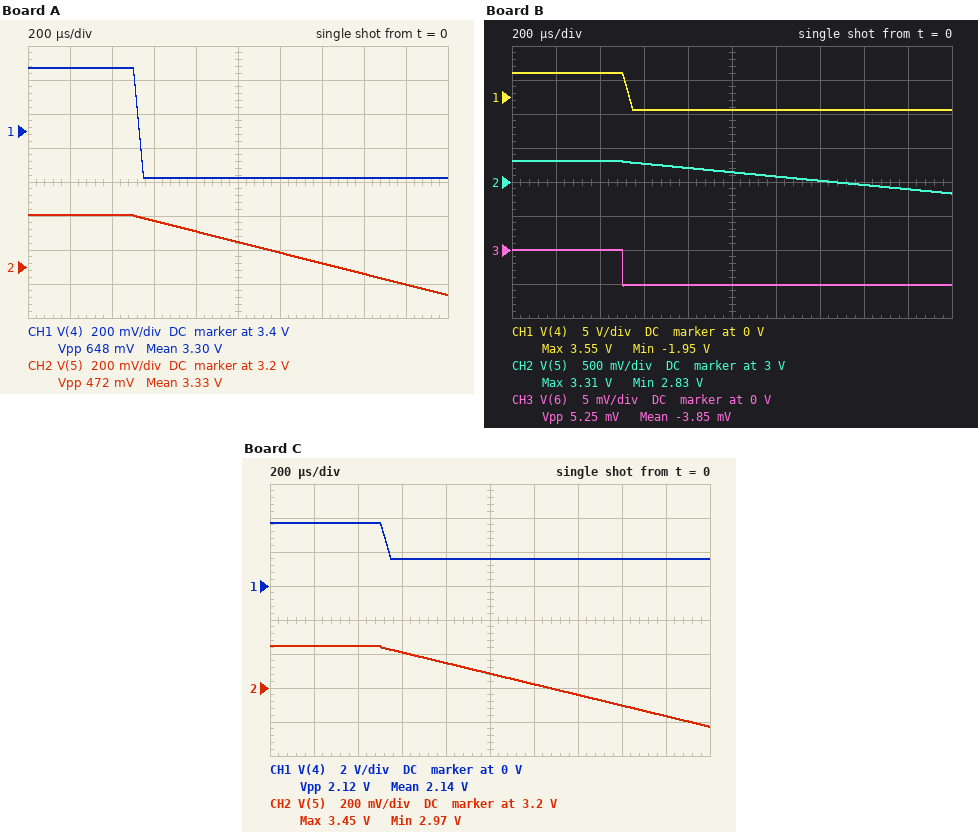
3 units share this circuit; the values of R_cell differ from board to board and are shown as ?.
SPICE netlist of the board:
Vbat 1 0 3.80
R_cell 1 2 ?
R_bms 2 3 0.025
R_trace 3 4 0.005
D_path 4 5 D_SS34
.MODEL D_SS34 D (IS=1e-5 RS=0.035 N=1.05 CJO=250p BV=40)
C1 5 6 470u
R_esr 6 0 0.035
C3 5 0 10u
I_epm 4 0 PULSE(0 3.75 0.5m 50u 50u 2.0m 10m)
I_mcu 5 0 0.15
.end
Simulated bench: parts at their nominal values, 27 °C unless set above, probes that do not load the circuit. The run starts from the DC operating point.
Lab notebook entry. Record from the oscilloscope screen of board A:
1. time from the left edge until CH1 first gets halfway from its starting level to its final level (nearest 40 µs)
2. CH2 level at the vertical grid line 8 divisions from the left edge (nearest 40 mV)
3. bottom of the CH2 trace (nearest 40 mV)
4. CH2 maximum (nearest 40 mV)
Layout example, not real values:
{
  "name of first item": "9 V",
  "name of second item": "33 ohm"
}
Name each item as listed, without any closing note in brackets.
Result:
{
  "time from the left edge until CH1 first gets halfway from its starting level to its final level": "520 µs",
  "CH2 level at the vertical grid line 8 divisions from the left edge": "3.16 V",
  "bottom of the CH2 trace": "3.04 V",
  "CH2 maximum": "3.52 V"
}
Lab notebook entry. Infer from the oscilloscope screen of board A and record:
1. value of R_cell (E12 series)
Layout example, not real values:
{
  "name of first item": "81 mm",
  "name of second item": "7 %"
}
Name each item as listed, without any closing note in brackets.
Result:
{
  "value of R_cell": "0.15 Ω"
}
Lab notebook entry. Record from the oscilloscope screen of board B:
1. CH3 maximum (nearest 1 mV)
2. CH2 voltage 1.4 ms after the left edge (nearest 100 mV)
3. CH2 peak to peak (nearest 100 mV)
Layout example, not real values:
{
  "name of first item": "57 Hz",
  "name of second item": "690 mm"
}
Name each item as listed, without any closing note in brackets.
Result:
{
  "CH3 maximum": "0 V",
  "CH2 voltage 1.4 ms after the left edge": "3.0 V",
  "CH2 peak to peak": "500 mV"
}
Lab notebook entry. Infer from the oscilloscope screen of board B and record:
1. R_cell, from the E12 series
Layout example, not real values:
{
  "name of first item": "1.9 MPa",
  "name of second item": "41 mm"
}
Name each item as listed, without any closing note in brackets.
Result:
{
  "R_cell, from the E12 series": "1.5 Ω"
}
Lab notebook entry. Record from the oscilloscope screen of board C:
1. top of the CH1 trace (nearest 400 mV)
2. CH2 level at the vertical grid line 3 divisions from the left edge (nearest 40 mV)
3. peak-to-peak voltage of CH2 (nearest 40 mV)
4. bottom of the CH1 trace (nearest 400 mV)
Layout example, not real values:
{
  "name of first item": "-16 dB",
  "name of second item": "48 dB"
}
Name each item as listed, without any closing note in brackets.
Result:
{
  "top of the CH1 trace": "3.6 V",
  "CH2 level at the vertical grid line 3 divisions from the left edge": "3.40 V",
  "peak-to-peak voltage of CH2": "480 mV",
  "bottom of the CH1 trace": "1.6 V"
}
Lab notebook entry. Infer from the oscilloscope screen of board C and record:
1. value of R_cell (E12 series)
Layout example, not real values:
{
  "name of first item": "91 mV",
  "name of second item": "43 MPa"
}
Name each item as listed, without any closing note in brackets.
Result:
{
  "value of R_cell": "0.56 Ω"
}
